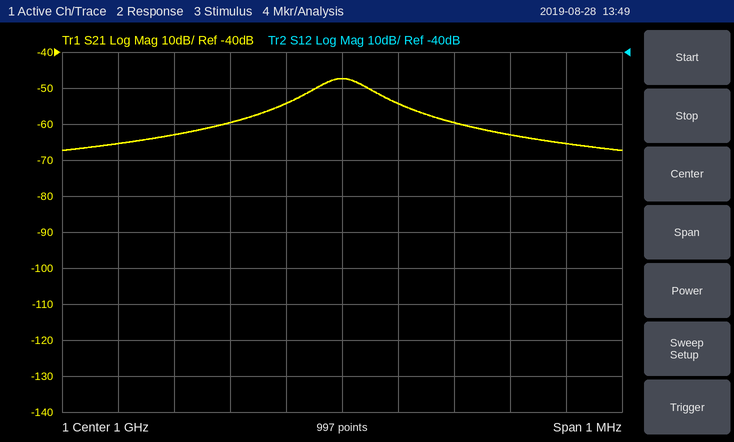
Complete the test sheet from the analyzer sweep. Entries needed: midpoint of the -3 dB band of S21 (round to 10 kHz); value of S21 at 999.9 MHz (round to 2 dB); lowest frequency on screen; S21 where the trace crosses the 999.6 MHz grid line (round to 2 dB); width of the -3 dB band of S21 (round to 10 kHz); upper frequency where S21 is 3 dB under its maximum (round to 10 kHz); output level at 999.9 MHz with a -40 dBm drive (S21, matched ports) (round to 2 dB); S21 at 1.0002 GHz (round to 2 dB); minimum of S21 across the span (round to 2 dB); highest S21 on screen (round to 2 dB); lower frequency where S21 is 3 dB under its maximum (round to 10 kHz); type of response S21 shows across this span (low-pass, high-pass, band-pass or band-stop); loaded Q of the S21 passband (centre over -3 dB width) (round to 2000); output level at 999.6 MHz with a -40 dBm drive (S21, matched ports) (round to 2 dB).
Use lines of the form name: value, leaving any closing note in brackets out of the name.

midpoint of the -3 dB band of S21: 1.00000 GHz
value of S21 at 999.9 MHz: -54 dB
lowest frequency on screen: 999.5 MHz
S21 where the trace crosses the 999.6 MHz grid line: -66 dB
width of the -3 dB band of S21: 100 kHz
upper frequency where S21 is 3 dB under its maximum: 1.00005 GHz
output level at 999.9 MHz with a -40 dBm drive (S21, matched ports): -94 dBm
S21 at 1.0002 GHz: -60 dB
minimum of S21 across the span: -68 dB
highest S21 on screen: -48 dB
lower frequency where S21 is 3 dB under its maximum: 999.95 MHz
type of response S21 shows across this span: band-pass
loaded Q of the S21 passband (centre over -3 dB width): 10000
output level at 999.6 MHz with a -40 dBm drive (S21, matched ports): -106 dBm
